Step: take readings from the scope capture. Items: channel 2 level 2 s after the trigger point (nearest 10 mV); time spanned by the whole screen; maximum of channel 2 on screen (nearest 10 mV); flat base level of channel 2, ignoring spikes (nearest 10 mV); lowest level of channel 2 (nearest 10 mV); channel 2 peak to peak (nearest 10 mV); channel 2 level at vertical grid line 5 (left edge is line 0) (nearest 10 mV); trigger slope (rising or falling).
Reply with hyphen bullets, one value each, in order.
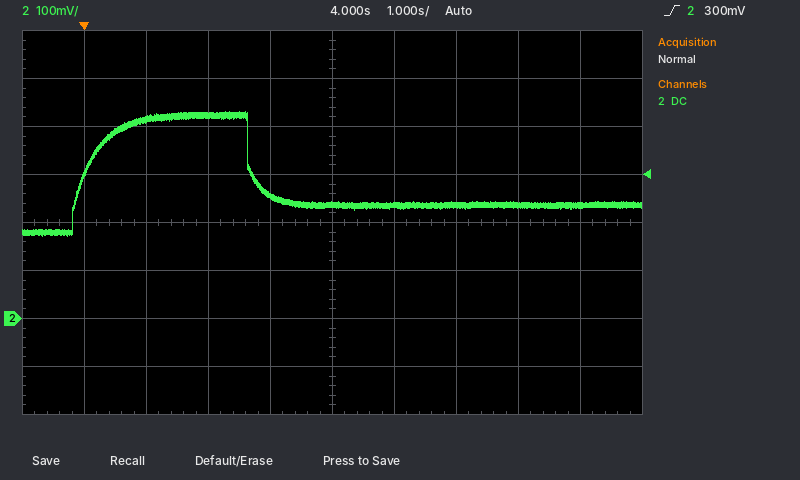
- 420 mV
- 10 s
- 430 mV
- 240 mV
- 170 mV
- 260 mV
- 240 mV
- rising
